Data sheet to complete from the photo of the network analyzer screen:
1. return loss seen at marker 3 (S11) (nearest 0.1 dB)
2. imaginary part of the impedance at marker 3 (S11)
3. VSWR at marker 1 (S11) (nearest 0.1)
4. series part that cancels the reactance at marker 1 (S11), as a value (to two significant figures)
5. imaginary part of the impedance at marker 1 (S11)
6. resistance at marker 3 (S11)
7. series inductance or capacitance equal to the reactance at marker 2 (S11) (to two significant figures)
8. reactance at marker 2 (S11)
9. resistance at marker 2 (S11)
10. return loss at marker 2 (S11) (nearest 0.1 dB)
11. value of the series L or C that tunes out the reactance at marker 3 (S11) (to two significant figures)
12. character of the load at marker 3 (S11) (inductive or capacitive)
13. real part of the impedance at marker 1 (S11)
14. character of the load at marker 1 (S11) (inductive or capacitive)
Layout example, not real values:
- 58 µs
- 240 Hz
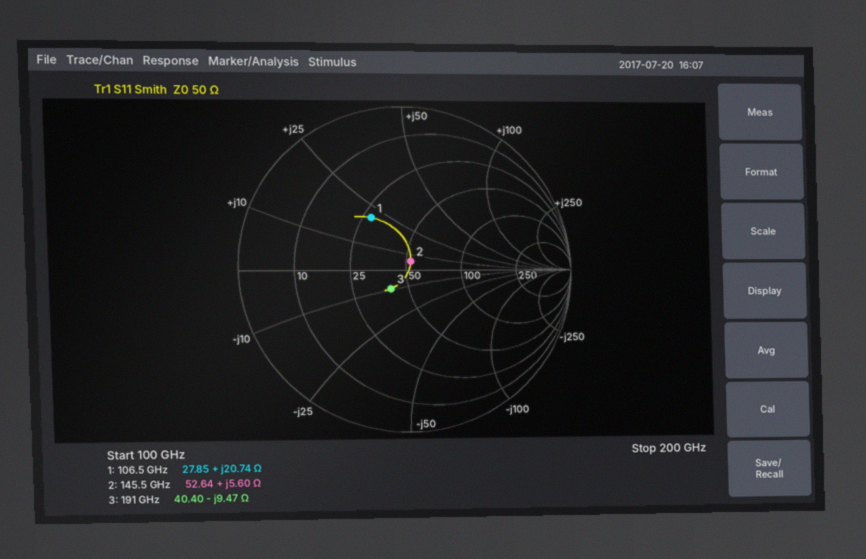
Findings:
- 16.6 dB
- -9.47 Ω
- 2.2
- 72 fF
- +20.74 Ω
- 40.40 Ω
- 6.1 pH
- +5.60 Ω
- 52.64 Ω
- 24.4 dB
- 7.9 pH
- capacitive
- 27.85 Ω
- inductive
